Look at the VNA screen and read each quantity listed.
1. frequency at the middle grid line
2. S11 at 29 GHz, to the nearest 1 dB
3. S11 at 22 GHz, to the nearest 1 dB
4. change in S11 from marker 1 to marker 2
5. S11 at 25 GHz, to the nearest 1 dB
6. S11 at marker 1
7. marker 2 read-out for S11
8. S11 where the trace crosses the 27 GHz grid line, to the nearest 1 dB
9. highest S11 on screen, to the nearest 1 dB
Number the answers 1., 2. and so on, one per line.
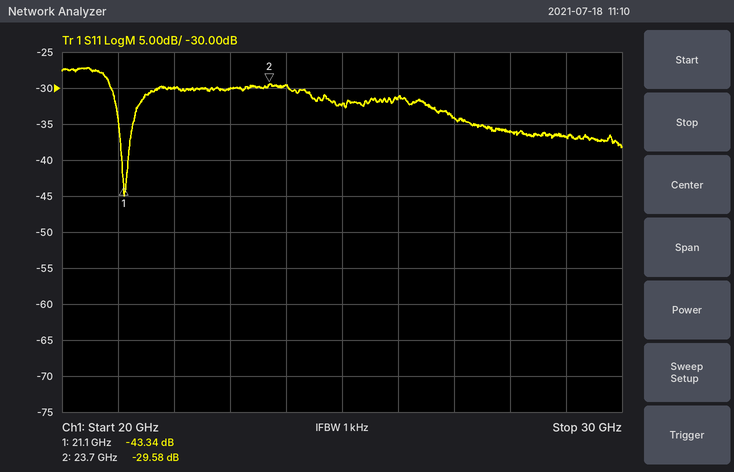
1. 25 GHz
2. -37 dB
3. -30 dB
4. 13.76 dB
5. -32 dB
6. -43.34 dB
7. -29.58 dB
8. -34 dB
9. -27 dB
